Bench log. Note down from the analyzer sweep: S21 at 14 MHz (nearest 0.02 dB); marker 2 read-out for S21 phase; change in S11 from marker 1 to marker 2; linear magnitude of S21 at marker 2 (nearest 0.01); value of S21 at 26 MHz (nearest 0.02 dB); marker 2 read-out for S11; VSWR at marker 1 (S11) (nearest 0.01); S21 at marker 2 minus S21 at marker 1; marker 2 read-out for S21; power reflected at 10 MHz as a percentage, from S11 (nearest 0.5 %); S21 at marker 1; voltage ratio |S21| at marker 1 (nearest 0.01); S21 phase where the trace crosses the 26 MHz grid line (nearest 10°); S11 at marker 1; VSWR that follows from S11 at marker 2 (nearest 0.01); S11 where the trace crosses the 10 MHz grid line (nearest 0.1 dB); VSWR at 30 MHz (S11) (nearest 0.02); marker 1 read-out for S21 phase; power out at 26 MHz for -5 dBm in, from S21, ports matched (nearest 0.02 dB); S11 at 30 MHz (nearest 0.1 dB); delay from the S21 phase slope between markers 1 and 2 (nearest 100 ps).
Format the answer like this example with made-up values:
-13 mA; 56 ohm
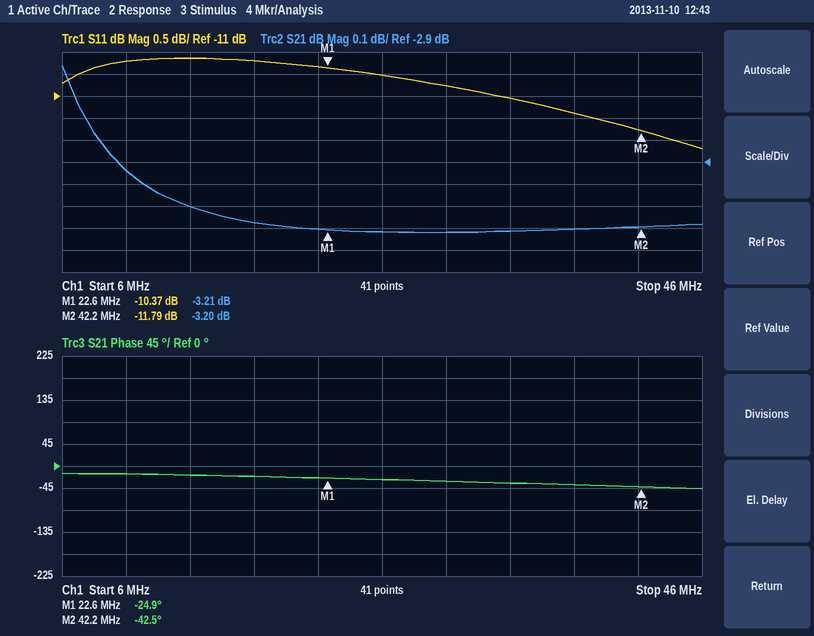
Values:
-3.10 dB; -42.5°; -1.42 dB; 0.69; -3.22 dB; -11.79 dB; 1.87; 0.01 dB; -3.20 dB; 9.5 %; -3.21 dB; 0.69; -30°; -10.37 dB; 1.69; -10.2 dB; 1.82; -24.9°; -8.22 dBm; -10.8 dB; 2.5 ns
